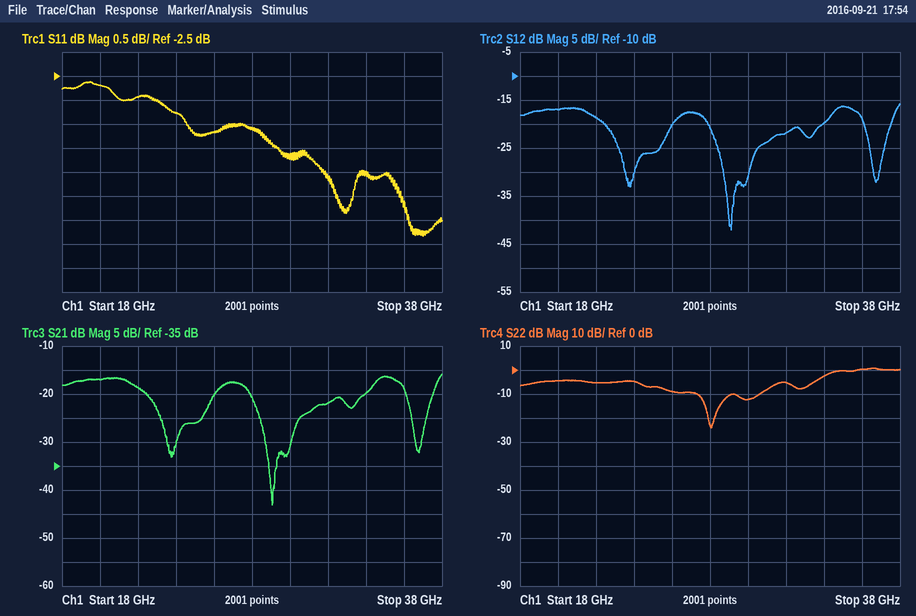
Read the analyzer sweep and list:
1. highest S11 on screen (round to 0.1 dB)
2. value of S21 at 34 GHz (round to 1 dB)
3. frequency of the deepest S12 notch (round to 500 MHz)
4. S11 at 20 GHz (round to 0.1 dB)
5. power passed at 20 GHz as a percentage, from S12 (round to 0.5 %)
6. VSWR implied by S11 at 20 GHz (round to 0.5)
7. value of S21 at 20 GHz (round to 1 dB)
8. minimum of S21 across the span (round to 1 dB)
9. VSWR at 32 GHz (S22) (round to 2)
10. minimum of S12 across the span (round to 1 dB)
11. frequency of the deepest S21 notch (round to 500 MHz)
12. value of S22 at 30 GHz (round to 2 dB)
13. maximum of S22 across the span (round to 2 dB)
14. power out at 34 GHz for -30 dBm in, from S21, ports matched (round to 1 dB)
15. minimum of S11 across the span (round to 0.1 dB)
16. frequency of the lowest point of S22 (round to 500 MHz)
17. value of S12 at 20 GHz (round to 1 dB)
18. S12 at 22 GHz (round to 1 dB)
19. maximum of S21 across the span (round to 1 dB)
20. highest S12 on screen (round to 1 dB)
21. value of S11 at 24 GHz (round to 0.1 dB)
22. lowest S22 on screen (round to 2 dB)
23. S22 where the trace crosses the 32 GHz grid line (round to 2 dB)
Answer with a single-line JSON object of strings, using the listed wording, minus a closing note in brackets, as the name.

{"highest S11 on screen": "-2.6 dB", "value of S21 at 34 GHz": "-20 dB", "frequency of the deepest S12 notch": "29.0 GHz", "S11 at 20 GHz": "-2.7 dB", "power passed at 20 GHz as a percentage, from S12": "2.0 %", "VSWR implied by S11 at 20 GHz": "6.5", "value of S21 at 20 GHz": "-17 dB", "minimum of S21 across the span": "-43 dB", "VSWR at 32 GHz (S22)": "4", "minimum of S12 across the span": "-42 dB", "frequency of the deepest S21 notch": "29.0 GHz", "value of S22 at 30 GHz": "-12 dB", "maximum of S22 across the span": "0 dB", "power out at 34 GHz for -30 dBm in, from S21, ports matched": "-50 dBm", "minimum of S11 across the span": "-5.8 dB", "frequency of the lowest point of S22": "28.0 GHz", "value of S12 at 20 GHz": "-17 dB", "S12 at 22 GHz": "-19 dB", "maximum of S21 across the span": "-16 dB", "highest S12 on screen": "-16 dB", "value of S11 at 24 GHz": "-3.3 dB", "lowest S22 on screen": "-24 dB", "S22 where the trace crosses the 32 GHz grid line": "-6 dB"}
